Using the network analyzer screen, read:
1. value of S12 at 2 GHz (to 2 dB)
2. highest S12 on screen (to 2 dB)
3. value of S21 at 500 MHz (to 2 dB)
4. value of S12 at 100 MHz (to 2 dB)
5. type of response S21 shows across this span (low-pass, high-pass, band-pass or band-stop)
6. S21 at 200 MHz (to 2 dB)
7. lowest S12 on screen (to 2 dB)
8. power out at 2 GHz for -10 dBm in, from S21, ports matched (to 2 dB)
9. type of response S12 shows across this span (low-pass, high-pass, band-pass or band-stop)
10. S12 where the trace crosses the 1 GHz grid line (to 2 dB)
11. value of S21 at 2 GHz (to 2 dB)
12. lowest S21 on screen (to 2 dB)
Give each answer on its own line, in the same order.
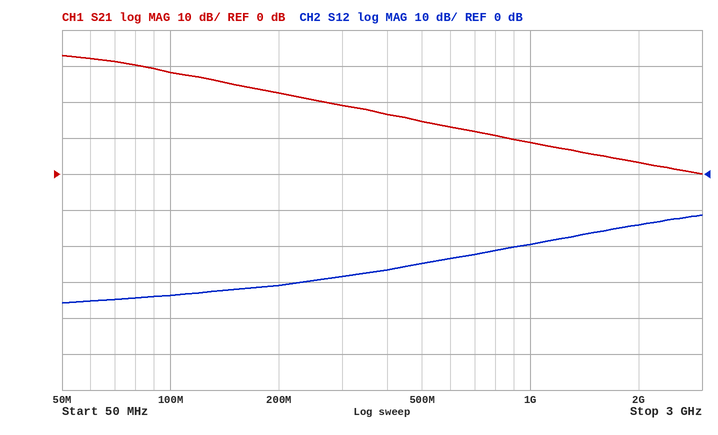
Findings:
-14 dB
-12 dB
14 dB
-34 dB
low-pass
22 dB
-36 dB
-6 dBm
high-pass
-20 dB
4 dB
0 dB
